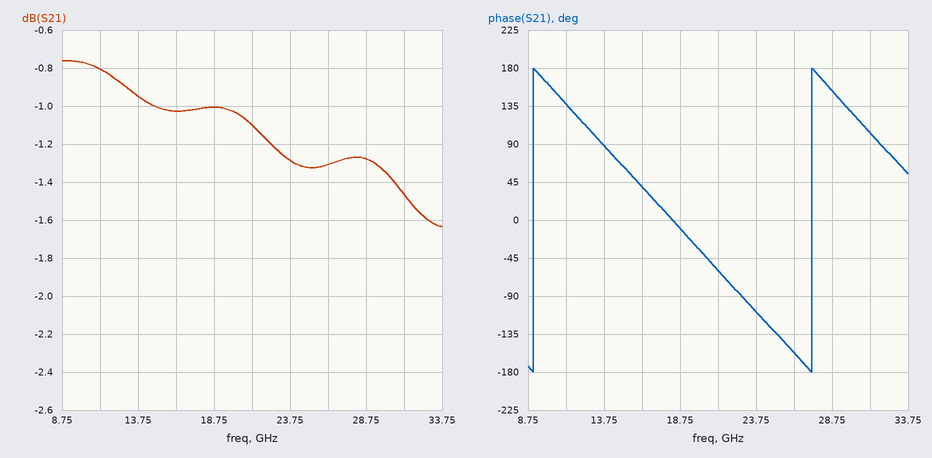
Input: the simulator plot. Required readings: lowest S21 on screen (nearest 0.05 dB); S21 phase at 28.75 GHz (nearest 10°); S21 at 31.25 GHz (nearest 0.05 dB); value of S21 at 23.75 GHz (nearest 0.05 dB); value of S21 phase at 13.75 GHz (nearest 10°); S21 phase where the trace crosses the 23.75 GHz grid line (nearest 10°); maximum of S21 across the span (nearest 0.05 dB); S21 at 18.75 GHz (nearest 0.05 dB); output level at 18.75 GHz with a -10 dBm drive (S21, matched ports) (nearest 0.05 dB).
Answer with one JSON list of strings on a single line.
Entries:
["-1.65 dB", "150°", "-1.45 dB", "-1.30 dB", "90°", "-110°", "-0.75 dB", "-1.00 dB", "-11.00 dBm"]
